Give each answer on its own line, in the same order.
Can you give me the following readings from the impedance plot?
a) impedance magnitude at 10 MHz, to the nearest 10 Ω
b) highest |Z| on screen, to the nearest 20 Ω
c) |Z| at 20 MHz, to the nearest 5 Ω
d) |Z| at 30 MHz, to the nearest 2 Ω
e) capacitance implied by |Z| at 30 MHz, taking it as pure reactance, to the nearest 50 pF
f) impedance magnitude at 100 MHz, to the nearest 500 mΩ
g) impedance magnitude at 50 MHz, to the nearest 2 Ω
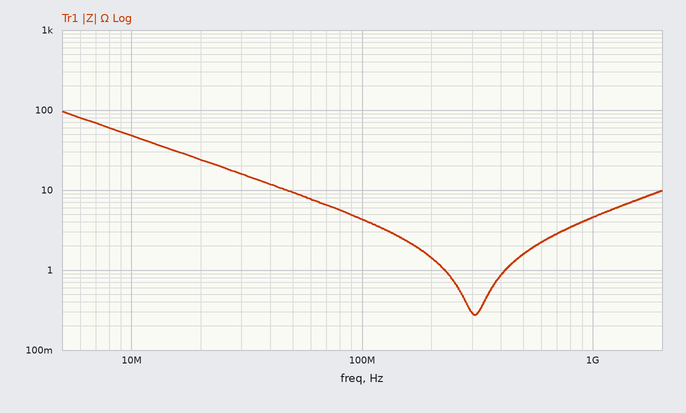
50 Ω
100 Ω
25 Ω
16 Ω
350 pF
4.5 Ω
10 Ω
